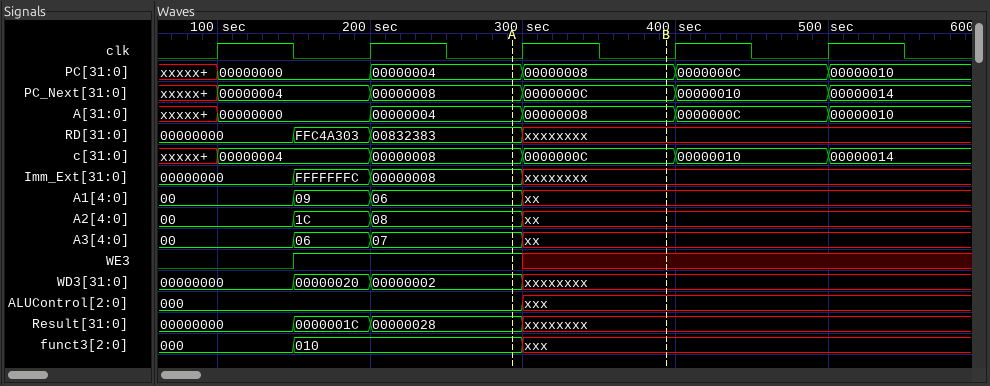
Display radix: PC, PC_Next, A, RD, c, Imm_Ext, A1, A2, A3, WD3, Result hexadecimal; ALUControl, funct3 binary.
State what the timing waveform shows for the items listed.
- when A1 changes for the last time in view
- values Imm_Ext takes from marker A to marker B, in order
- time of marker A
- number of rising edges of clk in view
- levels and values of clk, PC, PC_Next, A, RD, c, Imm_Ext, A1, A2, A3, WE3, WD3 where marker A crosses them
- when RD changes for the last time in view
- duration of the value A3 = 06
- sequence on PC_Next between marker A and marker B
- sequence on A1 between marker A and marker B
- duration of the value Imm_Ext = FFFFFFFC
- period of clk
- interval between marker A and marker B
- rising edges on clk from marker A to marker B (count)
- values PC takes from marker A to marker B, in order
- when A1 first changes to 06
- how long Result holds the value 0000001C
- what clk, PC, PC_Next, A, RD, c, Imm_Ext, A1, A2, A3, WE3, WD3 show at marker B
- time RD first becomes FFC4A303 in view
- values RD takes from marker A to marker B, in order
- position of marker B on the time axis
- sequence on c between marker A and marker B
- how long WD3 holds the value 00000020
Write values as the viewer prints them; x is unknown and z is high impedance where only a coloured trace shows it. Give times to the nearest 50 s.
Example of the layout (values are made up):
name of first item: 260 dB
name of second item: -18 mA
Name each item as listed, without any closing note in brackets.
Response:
when A1 changes for the last time in view: 300 s
values Imm_Ext takes from marker A to marker B, in order: 00000008, xxxxxxxx
time of marker A: 300 s
number of rising edges of clk in view: 5
levels and values of clk, PC, PC_Next, A, RD, c, Imm_Ext, A1, A2, A3, WE3, WD3 where marker A crosses them: clk=0, PC=00000004, PC_Next=00000008, A=00000004, RD=00832383, c=00000008, Imm_Ext=00000008, A1=06, A2=08, A3=07, WE3=1, WD3=00000002
when RD changes for the last time in view: 300 s
duration of the value A3 = 06: 50 s
sequence on PC_Next between marker A and marker B: 00000008, 0000000C
sequence on A1 between marker A and marker B: 06, xx
duration of the value Imm_Ext = FFFFFFFC: 50 s
period of clk: 100 s
interval between marker A and marker B: 100 s
rising edges on clk from marker A to marker B: 1
values PC takes from marker A to marker B, in order: 00000004, 00000008
when A1 first changes to 06: 200 s
how long Result holds the value 0000001C: 50 s
what clk, PC, PC_Next, A, RD, c, Imm_Ext, A1, A2, A3, WE3, WD3 show at marker B: clk=0, PC=00000008, PC_Next=0000000C, A=00000008, RD=xxxxxxxx, c=0000000C, Imm_Ext=xxxxxxxx, A1=xx, A2=xx, A3=xx, WE3=x, WD3=xxxxxxxx
time RD first becomes FFC4A303 in view: 150 s
values RD takes from marker A to marker B, in order: 00832383, xxxxxxxx
position of marker B on the time axis: 400 s
sequence on c between marker A and marker B: 00000008, 0000000C
how long WD3 holds the value 00000020: 50 s
